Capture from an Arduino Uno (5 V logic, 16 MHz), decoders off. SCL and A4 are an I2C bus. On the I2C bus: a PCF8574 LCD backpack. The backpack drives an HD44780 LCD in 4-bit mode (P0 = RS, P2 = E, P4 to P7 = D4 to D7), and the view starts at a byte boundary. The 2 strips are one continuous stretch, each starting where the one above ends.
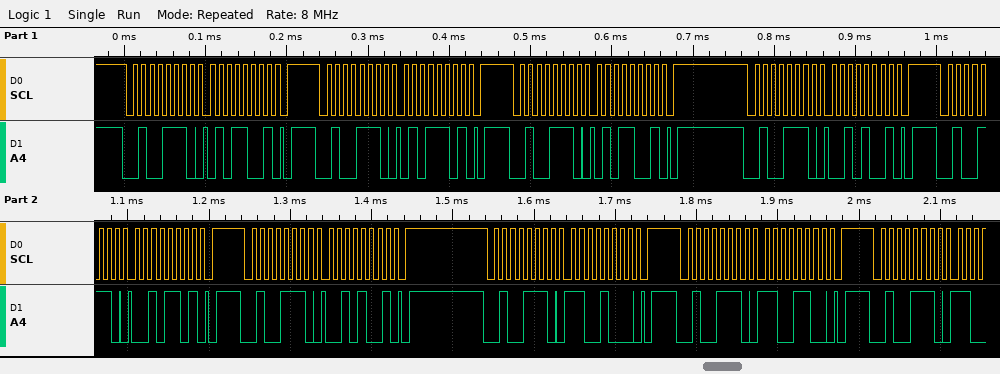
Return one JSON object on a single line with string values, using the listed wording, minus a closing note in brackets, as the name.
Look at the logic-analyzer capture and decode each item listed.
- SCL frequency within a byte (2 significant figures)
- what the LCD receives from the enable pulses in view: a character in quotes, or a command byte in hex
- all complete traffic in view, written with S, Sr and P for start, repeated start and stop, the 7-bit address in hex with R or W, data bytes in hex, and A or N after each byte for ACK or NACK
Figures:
{"SCL frequency within a byte": "100 kHz", "what the LCD receives from the enable pulses in view: a character in quotes, or a command byte in hex": "'R'", "all complete traffic in view, written with S, Sr and P for start, repeated start and stop, the 7-bit address in hex with R or W, data bytes in hex, and A or N after each byte for ACK or NACK": "S 27W A 59 A P S 27W A 5D A P S 27W A 59 A P S 27W A 29 A P S 27W A 2D A P S 27W A 29 A P S 27W A C8 A P S 27W A CC A P S 27W A"}
